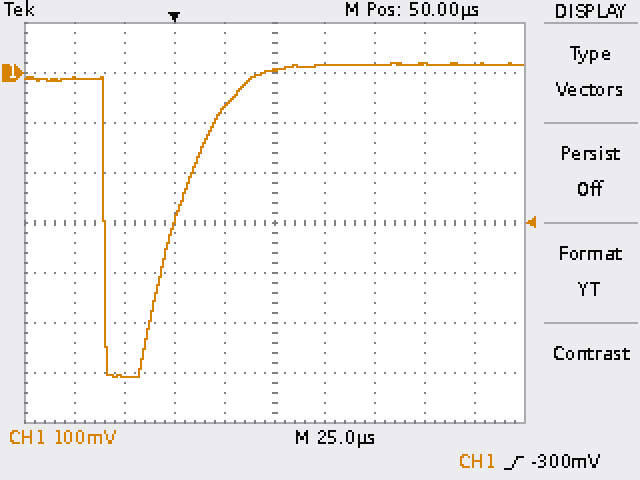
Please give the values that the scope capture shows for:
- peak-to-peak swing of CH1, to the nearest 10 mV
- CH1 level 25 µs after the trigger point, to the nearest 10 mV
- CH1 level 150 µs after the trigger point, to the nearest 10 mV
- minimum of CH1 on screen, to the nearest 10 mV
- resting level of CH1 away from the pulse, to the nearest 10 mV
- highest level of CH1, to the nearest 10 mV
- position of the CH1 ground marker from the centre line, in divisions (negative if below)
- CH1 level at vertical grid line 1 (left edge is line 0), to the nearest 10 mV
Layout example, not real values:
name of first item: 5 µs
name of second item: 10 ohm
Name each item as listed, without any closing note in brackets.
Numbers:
peak-to-peak swing of CH1, to the nearest 10 mV: 630 mV
CH1 level 25 µs after the trigger point, to the nearest 10 mV: -70 mV
CH1 level 150 µs after the trigger point, to the nearest 10 mV: 20 mV
minimum of CH1 on screen, to the nearest 10 mV: -610 mV
resting level of CH1 away from the pulse, to the nearest 10 mV: 20 mV
highest level of CH1, to the nearest 10 mV: 20 mV
position of the CH1 ground marker from the centre line, in divisions: +3.0 div
CH1 level at vertical grid line 1 (left edge is line 0), to the nearest 10 mV: -10 mV
